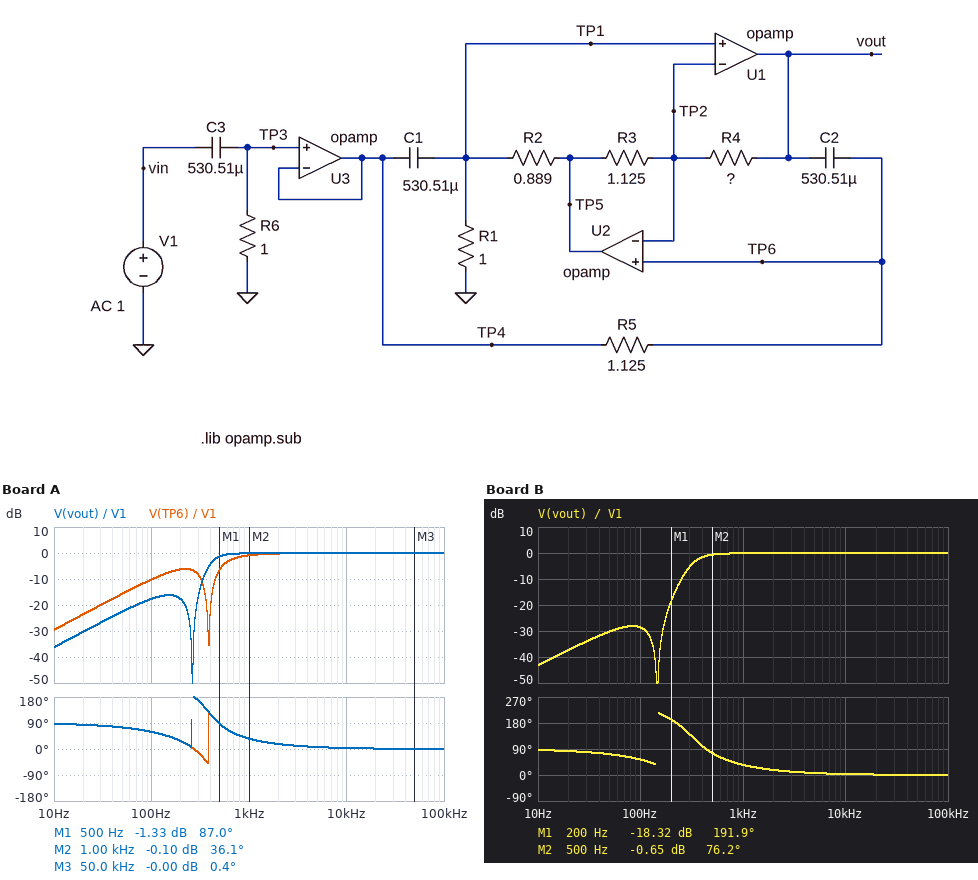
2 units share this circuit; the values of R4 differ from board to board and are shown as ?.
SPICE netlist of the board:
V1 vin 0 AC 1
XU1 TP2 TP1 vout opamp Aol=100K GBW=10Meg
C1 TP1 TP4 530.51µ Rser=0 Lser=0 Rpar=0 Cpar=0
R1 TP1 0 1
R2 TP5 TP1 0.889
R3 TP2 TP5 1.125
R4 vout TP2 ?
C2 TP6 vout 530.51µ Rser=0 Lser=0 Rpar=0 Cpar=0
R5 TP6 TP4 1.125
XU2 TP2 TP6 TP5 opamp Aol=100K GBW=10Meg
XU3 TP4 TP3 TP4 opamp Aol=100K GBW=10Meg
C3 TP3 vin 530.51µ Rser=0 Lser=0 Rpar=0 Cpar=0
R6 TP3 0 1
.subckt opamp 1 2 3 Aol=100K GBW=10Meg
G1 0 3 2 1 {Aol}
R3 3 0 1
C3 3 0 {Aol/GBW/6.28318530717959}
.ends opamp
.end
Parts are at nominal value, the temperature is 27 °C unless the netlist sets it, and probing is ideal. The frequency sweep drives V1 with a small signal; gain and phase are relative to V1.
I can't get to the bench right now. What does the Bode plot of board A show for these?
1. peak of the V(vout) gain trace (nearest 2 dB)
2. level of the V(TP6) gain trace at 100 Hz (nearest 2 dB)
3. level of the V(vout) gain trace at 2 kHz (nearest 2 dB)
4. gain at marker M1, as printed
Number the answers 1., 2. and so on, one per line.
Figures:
1. 0 dB
2. -10 dB
3. 0 dB
4. -1.33 dB
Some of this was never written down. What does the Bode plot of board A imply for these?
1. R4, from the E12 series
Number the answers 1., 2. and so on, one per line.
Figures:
1. 0.68 Ω
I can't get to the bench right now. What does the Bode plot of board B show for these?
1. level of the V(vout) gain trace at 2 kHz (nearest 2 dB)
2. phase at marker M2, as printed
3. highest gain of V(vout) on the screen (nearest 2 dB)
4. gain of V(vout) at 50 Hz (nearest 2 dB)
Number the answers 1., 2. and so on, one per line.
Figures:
1. 0 dB
2. 76.2 deg
3. 0 dB
4. -30 dB
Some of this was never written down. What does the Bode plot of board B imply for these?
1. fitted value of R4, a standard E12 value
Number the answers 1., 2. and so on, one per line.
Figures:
1. 1 Ω
